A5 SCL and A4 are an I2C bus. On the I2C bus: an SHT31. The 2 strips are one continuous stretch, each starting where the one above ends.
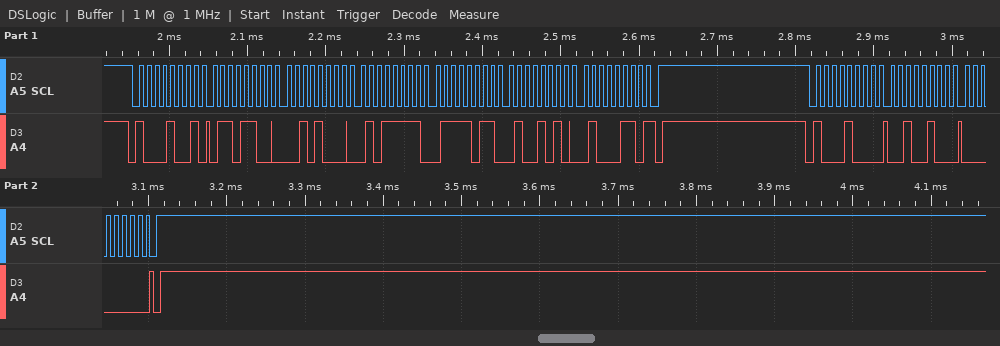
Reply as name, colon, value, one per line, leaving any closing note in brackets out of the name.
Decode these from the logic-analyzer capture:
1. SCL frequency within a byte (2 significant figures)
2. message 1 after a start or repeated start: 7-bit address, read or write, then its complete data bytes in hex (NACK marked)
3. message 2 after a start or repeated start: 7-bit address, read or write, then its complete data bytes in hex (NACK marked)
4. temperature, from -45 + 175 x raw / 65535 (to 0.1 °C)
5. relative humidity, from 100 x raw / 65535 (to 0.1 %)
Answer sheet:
SCL frequency within a byte: 100 kHz
message 1 after a start or repeated start: 7-bit address, read or write, then its complete data bytes in hex: 0x44 read: 6C 28 5F 7B 4A 46 NACK
message 2 after a start or repeated start: 7-bit address, read or write, then its complete data bytes in hex: 0x44 write: 24 00
temperature, from -45 + 175 x raw / 65535: 28.9 °C
relative humidity, from 100 x raw / 65535: 48.2 %
